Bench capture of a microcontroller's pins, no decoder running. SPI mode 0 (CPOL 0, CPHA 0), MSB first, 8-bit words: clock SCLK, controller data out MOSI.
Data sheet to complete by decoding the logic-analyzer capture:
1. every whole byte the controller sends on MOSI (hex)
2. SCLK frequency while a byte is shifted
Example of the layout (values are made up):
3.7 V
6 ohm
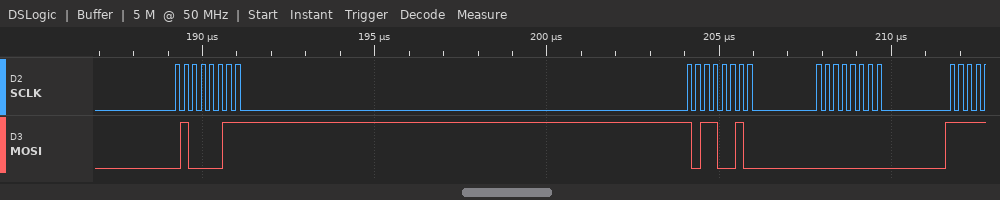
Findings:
0x43 0xB2 0x00
4 MHz
